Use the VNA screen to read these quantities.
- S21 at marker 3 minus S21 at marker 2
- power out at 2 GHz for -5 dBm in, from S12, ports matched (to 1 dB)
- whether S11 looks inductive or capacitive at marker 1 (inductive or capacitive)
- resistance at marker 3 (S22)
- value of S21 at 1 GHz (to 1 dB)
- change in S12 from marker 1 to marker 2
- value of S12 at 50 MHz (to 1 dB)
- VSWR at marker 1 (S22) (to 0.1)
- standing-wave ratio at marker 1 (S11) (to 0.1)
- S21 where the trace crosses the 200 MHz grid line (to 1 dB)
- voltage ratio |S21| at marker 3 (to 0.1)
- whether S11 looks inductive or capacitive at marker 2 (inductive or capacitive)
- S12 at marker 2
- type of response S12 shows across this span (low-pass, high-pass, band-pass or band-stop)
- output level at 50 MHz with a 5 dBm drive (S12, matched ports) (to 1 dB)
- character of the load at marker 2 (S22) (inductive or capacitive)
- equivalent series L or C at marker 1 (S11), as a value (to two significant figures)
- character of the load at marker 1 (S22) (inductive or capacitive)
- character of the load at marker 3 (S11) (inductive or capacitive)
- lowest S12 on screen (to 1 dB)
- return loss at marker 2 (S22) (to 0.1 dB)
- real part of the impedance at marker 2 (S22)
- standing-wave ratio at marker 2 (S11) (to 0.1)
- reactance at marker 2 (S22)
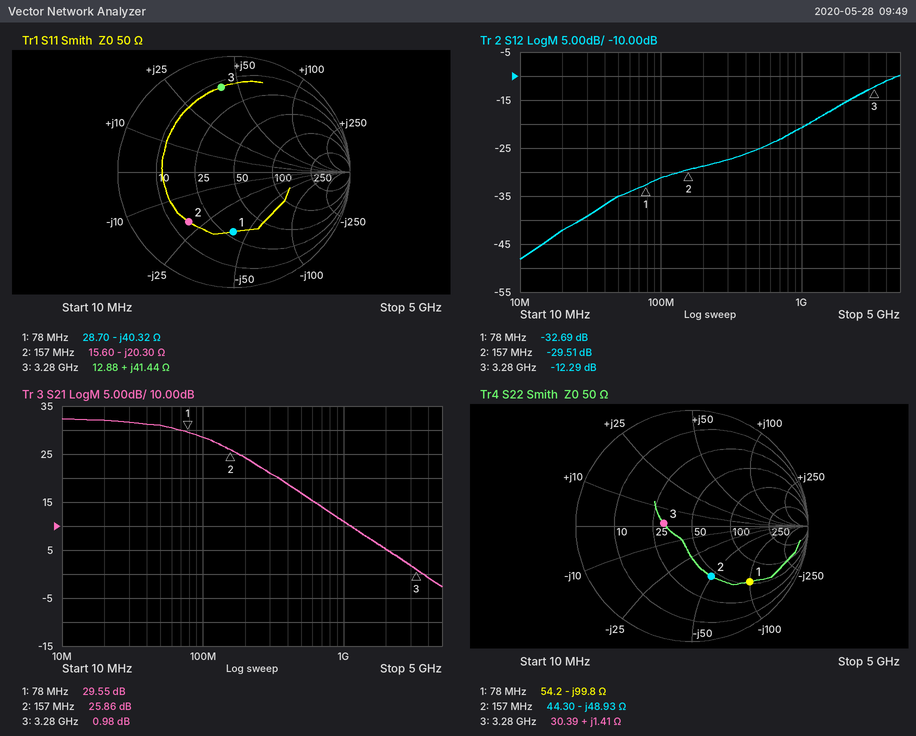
-24.88 dB
-21 dBm
capacitive
30.39 Ω
11 dB
3.18 dB
-35 dB
5.5
3.1
24 dB
1.1
capacitive
-29.51 dB
high-pass
-30 dBm
capacitive
51 pF
capacitive
inductive
-48 dB
6.7 dB
44.30 Ω
3.8
-48.93 Ω
